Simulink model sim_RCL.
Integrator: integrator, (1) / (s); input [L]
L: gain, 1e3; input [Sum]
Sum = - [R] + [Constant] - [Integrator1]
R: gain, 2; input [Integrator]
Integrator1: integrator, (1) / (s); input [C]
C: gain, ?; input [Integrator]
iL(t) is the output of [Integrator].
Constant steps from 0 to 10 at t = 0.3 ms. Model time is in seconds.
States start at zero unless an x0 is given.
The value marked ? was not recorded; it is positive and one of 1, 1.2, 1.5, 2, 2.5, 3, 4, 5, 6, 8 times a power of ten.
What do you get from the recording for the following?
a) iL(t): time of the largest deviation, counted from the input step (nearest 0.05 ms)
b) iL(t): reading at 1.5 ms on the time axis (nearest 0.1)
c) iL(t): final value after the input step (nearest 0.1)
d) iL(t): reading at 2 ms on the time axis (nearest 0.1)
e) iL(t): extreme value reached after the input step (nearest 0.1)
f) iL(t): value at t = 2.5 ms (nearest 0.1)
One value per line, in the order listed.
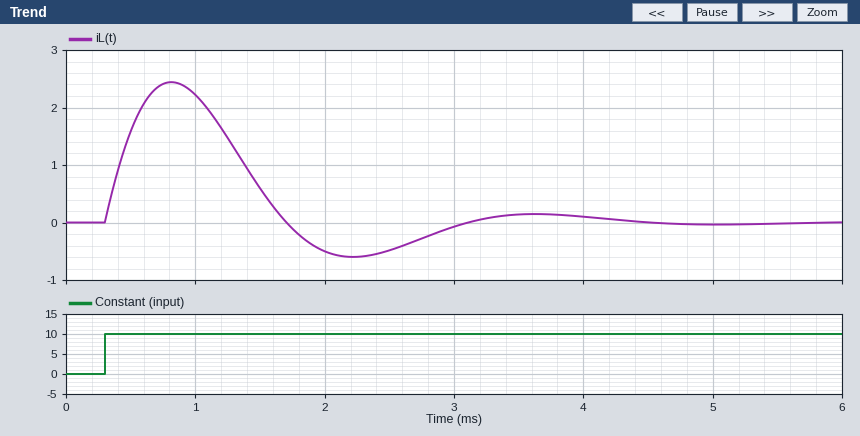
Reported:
0.50 ms
0.6
0.0
-0.5
2.4
-0.5
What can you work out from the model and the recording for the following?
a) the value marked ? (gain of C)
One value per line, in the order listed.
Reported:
6000
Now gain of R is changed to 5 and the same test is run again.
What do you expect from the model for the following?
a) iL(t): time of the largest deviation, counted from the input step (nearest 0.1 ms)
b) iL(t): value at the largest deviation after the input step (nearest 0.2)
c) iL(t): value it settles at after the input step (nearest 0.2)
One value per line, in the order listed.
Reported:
0.4 ms
1.4
0.0
